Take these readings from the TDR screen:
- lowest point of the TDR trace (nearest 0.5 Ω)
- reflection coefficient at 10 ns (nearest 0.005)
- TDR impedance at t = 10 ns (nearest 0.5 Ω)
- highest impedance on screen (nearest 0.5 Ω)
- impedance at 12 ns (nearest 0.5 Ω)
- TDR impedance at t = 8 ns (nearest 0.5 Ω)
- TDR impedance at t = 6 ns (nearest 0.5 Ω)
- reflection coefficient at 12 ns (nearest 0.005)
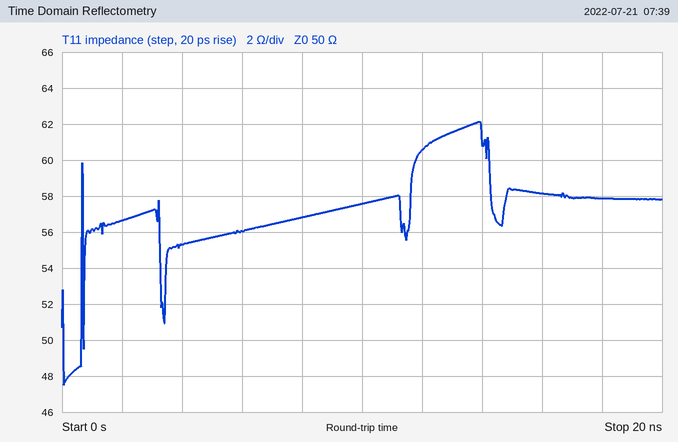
47.5 Ω
+0.070
57.5 Ω
62.0 Ω
60.5 Ω
57.0 Ω
56.0 Ω
+0.095
